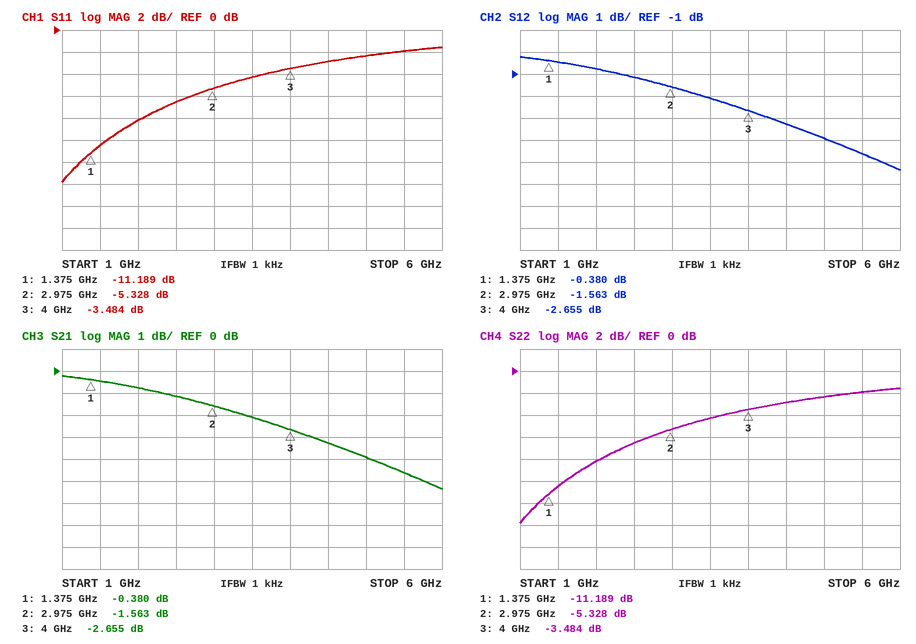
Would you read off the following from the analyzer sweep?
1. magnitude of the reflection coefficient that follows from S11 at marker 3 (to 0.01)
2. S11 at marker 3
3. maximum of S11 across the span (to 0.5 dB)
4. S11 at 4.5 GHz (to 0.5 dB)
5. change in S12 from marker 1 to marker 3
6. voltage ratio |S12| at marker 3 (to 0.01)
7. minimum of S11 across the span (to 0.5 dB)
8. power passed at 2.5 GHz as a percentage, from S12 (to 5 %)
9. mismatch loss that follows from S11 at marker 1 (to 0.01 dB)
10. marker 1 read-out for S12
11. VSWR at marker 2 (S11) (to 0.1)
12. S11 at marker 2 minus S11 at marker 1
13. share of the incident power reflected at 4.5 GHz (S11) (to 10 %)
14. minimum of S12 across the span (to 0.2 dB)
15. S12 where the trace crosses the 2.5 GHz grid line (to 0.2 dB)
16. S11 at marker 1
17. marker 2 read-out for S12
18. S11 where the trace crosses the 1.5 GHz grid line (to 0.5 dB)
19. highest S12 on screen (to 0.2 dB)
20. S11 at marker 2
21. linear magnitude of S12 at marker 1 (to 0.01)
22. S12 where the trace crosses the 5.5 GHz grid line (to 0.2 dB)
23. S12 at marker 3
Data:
0.67
-3.484 dB
-1.5 dB
-3.0 dB
-2.275 dB
0.74
-14.0 dB
75 %
0.34 dB
-0.380 dB
3.4
5.861 dB
50 %
-5.4 dB
-1.2 dB
-11.189 dB
-1.563 dB
-10.5 dB
-0.2 dB
-5.328 dB
0.96
-4.6 dB
-2.655 dB
